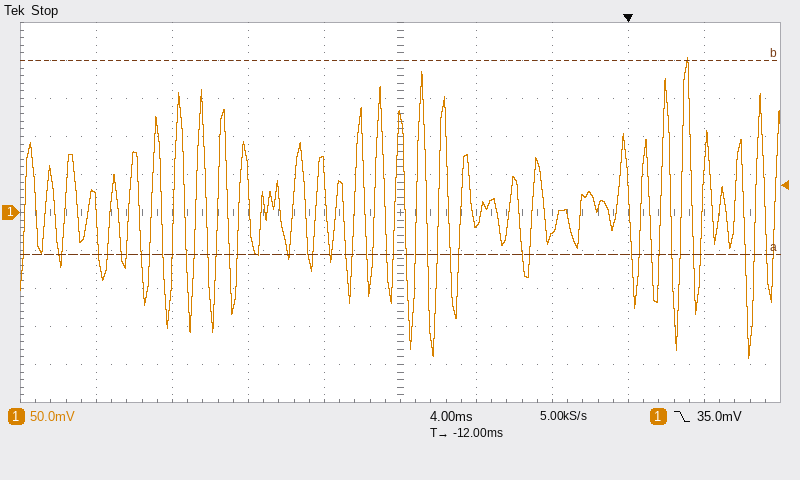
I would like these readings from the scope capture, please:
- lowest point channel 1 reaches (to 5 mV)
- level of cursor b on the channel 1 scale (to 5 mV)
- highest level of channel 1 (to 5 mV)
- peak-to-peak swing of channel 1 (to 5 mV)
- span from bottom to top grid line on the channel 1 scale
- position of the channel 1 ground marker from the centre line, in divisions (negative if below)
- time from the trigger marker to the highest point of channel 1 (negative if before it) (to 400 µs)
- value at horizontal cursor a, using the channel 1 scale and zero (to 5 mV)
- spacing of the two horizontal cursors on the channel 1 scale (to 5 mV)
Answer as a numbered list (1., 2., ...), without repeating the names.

1. -190 mV
2. 200 mV
3. 205 mV
4. 395 mV
5. 500 mV
6. 0.0 div
7. +3.2 ms
8. -55 mV
9. 255 mV
